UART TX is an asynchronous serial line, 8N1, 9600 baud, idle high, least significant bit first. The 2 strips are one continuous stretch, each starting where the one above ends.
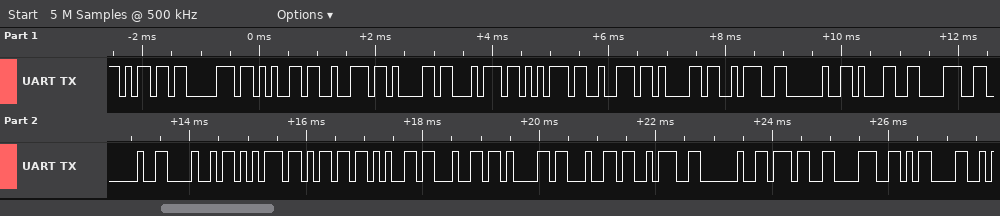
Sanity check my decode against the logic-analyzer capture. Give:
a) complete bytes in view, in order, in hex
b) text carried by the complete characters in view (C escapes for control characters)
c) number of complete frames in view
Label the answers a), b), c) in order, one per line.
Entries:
a) 0x6D 0x70 0x65 0x72 0x61 0x74 0x75 0x72 0x61 0x3A 0x20 0x31 0x38 0x20 0x48 0x75 0x6D 0x65 0x64 0x61 0x64 0x3A 0x20 0x37 0x38 0x0D
b) "mperatura: 18 Humedad: 78\r"
c) 26
